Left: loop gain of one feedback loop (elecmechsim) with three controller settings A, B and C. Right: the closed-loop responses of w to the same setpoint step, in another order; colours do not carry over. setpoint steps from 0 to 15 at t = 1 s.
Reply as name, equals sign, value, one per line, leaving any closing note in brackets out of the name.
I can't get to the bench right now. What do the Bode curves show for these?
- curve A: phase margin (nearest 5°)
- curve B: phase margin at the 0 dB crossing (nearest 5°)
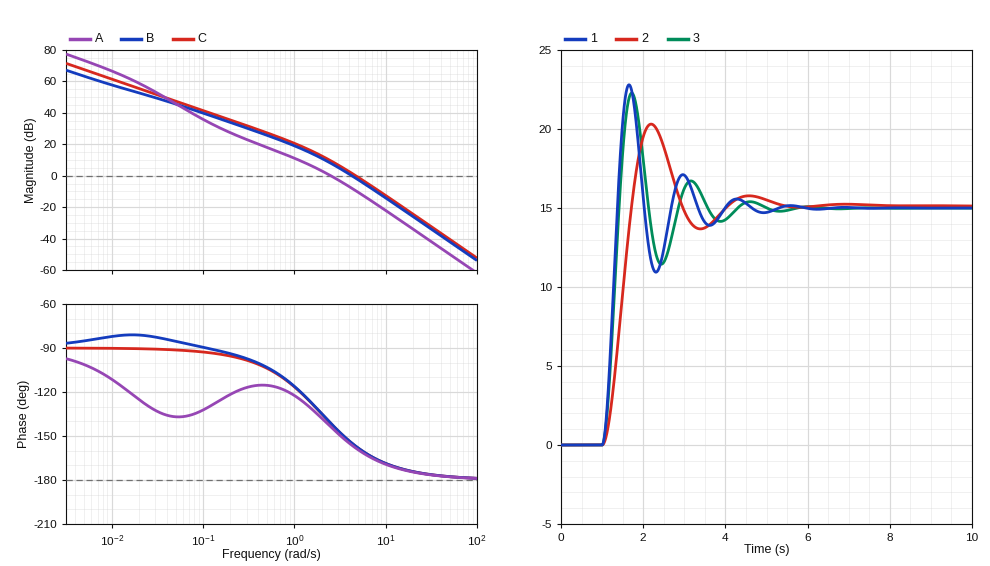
curve A: phase margin = 35°
curve B: phase margin at the 0 dB crossing = 25°
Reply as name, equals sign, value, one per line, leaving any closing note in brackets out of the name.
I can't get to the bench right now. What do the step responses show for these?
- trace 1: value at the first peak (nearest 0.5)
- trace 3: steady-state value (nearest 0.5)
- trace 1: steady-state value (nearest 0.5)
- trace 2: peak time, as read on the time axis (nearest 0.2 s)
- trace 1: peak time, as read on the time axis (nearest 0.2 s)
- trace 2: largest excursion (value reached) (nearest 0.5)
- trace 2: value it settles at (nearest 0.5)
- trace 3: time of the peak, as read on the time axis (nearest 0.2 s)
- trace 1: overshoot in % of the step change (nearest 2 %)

trace 1: value at the first peak = 23.0
trace 3: steady-state value = 15.0
trace 1: steady-state value = 15.0
trace 2: peak time, as read on the time axis = 2.2 s
trace 1: peak time, as read on the time axis = 1.6 s
trace 2: largest excursion (value reached) = 20.5
trace 2: value it settles at = 15.0
trace 3: time of the peak, as read on the time axis = 1.8 s
trace 1: overshoot in % of the step change = 52 %
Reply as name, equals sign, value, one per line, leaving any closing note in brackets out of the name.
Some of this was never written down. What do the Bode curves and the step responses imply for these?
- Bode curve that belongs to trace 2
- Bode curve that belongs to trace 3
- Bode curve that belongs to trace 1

Bode curve that belongs to trace 2 = A
Bode curve that belongs to trace 3 = B
Bode curve that belongs to trace 1 = C
